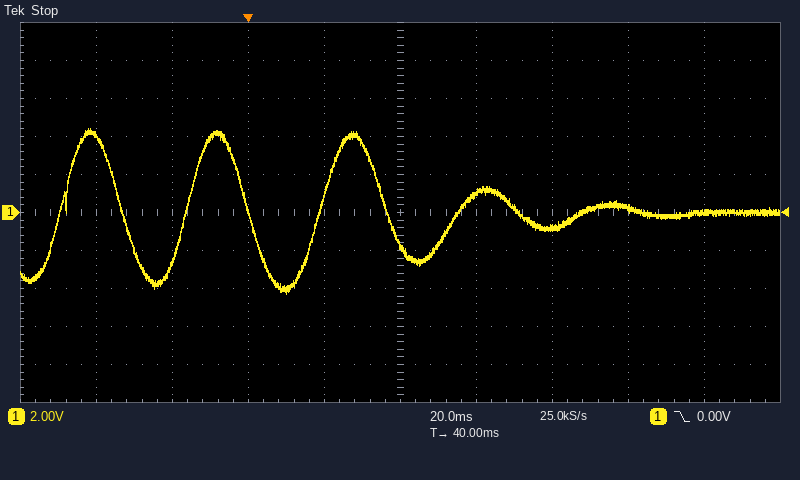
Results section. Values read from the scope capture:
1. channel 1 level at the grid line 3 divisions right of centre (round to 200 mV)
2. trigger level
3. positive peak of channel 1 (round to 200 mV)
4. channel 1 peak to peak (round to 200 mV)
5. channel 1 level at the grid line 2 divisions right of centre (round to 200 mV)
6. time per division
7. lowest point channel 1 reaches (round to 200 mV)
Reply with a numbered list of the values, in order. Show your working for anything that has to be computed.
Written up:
1. 200 mV
2. 0.00 V
3. 4.4 V
4. 4.4 V − (-4.2 V) = 8.6 V
5. -800 mV
6. 20 ms
7. -4.2 V
